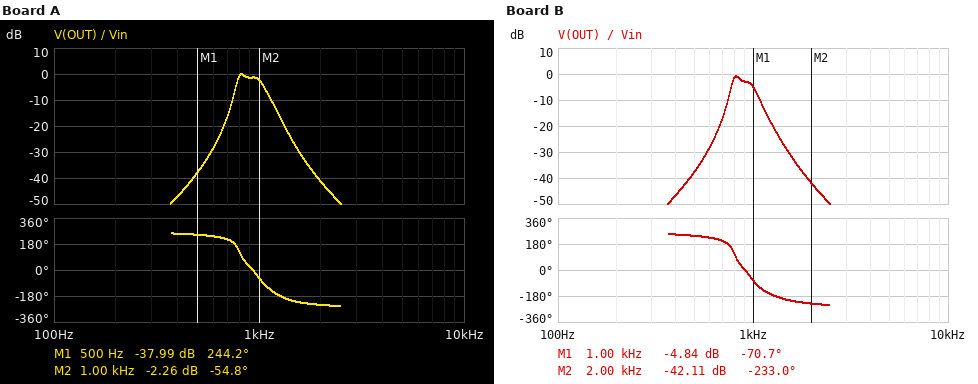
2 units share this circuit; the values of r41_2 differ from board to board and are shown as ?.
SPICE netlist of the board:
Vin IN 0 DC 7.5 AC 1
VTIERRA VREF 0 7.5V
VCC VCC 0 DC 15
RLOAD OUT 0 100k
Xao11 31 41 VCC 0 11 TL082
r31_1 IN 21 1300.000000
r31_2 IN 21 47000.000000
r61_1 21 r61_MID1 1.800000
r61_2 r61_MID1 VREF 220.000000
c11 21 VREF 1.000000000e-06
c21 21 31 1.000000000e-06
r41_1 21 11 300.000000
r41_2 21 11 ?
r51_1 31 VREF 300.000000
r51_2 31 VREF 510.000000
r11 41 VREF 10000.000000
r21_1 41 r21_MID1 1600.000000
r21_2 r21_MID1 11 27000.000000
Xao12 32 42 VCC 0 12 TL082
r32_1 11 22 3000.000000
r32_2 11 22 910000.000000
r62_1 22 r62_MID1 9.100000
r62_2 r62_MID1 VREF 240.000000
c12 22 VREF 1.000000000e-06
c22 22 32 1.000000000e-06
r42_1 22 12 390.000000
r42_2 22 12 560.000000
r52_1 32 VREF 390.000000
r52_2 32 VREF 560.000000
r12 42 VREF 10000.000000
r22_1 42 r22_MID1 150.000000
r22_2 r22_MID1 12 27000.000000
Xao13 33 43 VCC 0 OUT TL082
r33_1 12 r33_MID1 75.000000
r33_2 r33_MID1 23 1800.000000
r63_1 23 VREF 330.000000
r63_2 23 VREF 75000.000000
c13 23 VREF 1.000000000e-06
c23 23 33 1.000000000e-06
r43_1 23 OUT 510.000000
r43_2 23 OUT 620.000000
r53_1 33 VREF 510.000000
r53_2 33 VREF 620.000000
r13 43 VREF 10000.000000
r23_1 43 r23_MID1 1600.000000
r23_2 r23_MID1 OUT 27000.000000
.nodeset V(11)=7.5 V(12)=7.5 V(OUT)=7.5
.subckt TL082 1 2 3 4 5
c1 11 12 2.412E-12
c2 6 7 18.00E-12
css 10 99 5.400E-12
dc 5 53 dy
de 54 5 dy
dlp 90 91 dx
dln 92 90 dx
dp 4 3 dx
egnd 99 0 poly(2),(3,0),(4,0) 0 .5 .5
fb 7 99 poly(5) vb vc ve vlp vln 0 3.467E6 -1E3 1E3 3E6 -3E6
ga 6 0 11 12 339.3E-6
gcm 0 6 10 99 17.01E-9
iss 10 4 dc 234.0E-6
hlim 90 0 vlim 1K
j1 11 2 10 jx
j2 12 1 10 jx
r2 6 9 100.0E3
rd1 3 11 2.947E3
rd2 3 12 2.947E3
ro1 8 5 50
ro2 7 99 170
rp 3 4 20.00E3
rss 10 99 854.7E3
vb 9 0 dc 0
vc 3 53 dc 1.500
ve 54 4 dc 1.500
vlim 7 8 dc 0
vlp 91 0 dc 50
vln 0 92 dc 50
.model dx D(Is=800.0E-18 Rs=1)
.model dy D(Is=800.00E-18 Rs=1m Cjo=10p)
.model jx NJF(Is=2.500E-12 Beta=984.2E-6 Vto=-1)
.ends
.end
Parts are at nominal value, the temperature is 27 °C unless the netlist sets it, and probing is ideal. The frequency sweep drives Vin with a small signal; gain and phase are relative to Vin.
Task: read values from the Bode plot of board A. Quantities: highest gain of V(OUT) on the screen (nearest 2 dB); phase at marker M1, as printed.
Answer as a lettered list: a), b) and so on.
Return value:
a) 0 dB
b) 244.2 deg
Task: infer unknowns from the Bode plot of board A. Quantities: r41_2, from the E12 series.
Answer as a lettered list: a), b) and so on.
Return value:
a) 820 Ω
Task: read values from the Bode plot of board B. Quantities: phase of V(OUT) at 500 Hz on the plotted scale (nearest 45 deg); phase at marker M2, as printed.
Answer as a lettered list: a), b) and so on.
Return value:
a) 225 deg
b) -233.0 deg
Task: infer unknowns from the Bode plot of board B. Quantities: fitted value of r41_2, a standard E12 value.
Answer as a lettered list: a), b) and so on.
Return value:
a) 1.5 kΩ
